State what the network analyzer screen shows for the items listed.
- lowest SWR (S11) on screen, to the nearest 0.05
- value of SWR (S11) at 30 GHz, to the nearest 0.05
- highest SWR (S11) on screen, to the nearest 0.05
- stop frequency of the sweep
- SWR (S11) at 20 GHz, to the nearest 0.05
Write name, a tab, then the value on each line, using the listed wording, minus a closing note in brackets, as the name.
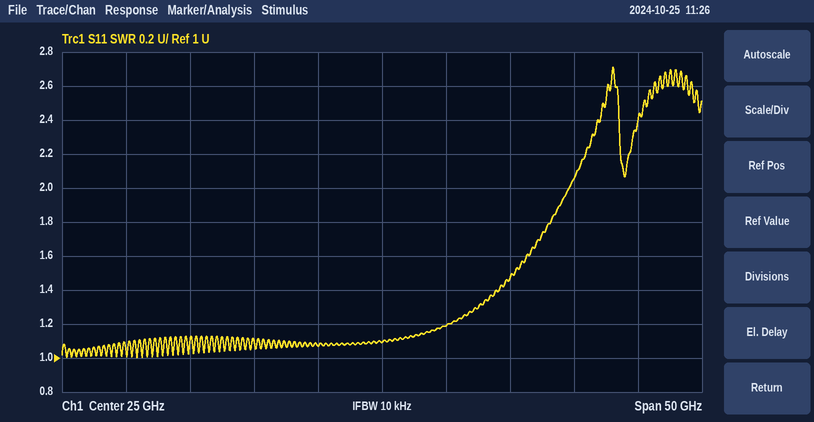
lowest SWR (S11) on screen, to the nearest 0.05	1.00
value of SWR (S11) at 30 GHz, to the nearest 0.05	1.20
highest SWR (S11) on screen, to the nearest 0.05	2.70
stop frequency of the sweep	50 GHz
SWR (S11) at 20 GHz, to the nearest 0.05	1.05
